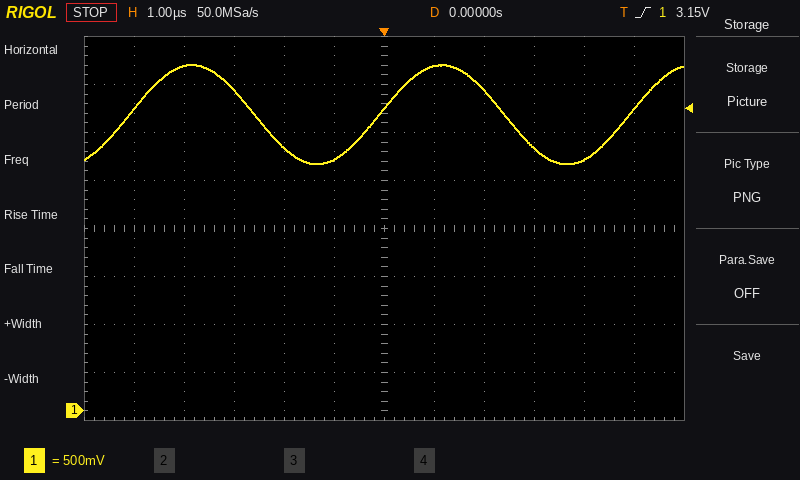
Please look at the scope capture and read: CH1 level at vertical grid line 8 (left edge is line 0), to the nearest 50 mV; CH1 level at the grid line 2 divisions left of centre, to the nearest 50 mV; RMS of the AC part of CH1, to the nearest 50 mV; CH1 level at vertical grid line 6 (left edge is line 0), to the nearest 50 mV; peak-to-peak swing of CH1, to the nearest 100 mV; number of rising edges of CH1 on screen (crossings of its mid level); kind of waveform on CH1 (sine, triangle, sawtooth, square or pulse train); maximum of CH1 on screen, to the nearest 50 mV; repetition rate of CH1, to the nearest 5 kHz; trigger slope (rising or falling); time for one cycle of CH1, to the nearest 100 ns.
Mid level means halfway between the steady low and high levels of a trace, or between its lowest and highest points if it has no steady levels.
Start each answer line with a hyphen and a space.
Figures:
- 3.35 V
- 2.75 V
- 350 mV
- 3.15 V
- 1.00 V
- 3
- sine
- 3.60 V
- 200 kHz
- rising
- 5.0 µs
